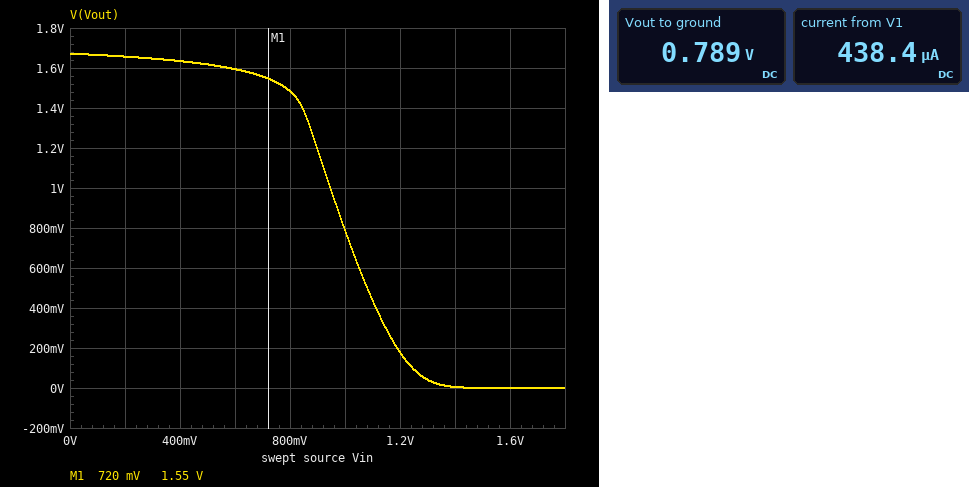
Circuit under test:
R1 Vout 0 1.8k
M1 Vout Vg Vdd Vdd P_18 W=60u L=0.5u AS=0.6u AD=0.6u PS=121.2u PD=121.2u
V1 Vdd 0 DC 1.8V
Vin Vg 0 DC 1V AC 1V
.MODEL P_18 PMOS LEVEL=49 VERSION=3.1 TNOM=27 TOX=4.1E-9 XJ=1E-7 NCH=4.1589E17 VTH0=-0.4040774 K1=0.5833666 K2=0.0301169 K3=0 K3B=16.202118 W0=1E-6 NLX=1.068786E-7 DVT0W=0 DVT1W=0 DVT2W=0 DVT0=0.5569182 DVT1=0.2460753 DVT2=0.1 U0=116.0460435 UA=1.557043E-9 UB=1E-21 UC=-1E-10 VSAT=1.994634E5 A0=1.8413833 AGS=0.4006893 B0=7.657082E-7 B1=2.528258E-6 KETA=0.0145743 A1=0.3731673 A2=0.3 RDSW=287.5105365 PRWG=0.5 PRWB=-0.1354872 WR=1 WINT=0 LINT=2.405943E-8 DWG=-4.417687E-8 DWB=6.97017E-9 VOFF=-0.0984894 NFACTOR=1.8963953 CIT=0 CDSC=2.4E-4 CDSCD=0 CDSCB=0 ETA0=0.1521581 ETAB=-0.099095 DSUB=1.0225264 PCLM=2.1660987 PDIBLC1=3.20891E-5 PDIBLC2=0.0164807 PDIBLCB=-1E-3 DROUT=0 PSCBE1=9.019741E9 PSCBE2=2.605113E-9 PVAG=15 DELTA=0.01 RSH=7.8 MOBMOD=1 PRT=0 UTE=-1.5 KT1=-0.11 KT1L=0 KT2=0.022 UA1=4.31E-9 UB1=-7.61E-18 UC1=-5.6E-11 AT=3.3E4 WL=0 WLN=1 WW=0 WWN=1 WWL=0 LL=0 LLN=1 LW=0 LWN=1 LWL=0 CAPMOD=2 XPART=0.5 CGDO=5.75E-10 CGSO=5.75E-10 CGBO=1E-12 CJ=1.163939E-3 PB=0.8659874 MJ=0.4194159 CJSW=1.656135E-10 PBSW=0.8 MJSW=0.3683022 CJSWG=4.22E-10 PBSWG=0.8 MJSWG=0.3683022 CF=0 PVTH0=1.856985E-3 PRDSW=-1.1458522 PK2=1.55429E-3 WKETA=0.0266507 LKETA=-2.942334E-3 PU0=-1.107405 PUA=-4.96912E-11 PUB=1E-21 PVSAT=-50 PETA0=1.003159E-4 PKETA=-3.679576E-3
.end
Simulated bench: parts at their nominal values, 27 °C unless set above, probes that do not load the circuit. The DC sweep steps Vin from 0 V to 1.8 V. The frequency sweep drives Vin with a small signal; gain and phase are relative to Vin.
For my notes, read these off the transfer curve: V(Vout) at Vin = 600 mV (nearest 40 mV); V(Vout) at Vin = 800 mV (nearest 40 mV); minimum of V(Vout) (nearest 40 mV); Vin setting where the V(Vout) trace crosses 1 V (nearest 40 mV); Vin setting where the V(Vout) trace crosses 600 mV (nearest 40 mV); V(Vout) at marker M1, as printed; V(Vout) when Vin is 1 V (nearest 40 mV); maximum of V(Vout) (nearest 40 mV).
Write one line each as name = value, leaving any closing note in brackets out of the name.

V(Vout) at Vin = 600 mV = 1.60 V
V(Vout) at Vin = 800 mV = 1.48 V
minimum of V(Vout) = 0 V
Vin setting where the V(Vout) trace crosses 1 V = 960 mV
Vin setting where the V(Vout) trace crosses 600 mV = 1.04 V
V(Vout) at marker M1, as printed = 1.55 V
V(Vout) when Vin is 1 V = 800 mV
maximum of V(Vout) = 1.68 V
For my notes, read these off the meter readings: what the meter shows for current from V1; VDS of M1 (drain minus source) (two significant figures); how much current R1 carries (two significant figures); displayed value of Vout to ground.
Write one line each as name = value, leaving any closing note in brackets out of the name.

what the meter shows for current from V1 = 438.4 µA
VDS of M1 (drain minus source) = -1.0 V
how much current R1 carries = 440 µA
displayed value of Vout to ground = 0.789 V
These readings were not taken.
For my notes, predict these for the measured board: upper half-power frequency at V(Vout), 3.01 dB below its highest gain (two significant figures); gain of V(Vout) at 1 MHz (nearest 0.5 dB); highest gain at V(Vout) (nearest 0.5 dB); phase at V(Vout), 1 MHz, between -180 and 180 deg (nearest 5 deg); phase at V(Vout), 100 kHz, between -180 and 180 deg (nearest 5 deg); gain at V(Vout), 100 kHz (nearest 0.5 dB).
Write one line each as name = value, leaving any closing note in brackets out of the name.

upper half-power frequency at V(Vout), 3.01 dB below its highest gain = 180 kHz
gain of V(Vout) at 1 MHz = -3.0 dB
highest gain at V(Vout) = 11.5 dB
phase at V(Vout), 1 MHz, between -180 and 180 deg = 100 deg
phase at V(Vout), 100 kHz, between -180 and 180 deg = 150 deg
gain at V(Vout), 100 kHz = 10.5 dB
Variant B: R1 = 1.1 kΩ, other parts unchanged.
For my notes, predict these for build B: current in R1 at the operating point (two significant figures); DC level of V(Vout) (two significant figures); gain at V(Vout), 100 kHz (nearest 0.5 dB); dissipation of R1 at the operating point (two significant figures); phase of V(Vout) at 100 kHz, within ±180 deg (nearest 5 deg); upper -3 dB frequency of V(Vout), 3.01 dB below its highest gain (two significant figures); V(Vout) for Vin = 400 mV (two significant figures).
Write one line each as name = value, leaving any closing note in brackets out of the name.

current in R1 at the operating point = 450 µA
DC level of V(Vout) = 490 mV
gain at V(Vout), 100 kHz = 7.5 dB
dissipation of R1 at the operating point = 220 µW
phase of V(Vout) at 100 kHz, within ±180 deg = 160 deg
upper -3 dB frequency of V(Vout), 3.01 dB below its highest gain = 310 kHz
V(Vout) for Vin = 400 mV = 1.5 V
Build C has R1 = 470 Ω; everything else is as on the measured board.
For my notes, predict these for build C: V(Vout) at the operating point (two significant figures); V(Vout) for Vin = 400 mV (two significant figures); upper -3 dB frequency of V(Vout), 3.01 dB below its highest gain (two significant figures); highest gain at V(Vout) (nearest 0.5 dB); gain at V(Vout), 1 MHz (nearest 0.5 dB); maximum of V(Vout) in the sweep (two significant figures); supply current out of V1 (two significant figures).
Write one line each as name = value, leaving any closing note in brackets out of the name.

V(Vout) at the operating point = 210 mV
V(Vout) for Vin = 400 mV = 1.1 V
upper -3 dB frequency of V(Vout), 3.01 dB below its highest gain = 750 kHz
highest gain at V(Vout) = 0.5 dB
gain at V(Vout), 1 MHz = -4.0 dB
maximum of V(Vout) in the sweep = 1.3 V
supply current out of V1 = 450 µA
